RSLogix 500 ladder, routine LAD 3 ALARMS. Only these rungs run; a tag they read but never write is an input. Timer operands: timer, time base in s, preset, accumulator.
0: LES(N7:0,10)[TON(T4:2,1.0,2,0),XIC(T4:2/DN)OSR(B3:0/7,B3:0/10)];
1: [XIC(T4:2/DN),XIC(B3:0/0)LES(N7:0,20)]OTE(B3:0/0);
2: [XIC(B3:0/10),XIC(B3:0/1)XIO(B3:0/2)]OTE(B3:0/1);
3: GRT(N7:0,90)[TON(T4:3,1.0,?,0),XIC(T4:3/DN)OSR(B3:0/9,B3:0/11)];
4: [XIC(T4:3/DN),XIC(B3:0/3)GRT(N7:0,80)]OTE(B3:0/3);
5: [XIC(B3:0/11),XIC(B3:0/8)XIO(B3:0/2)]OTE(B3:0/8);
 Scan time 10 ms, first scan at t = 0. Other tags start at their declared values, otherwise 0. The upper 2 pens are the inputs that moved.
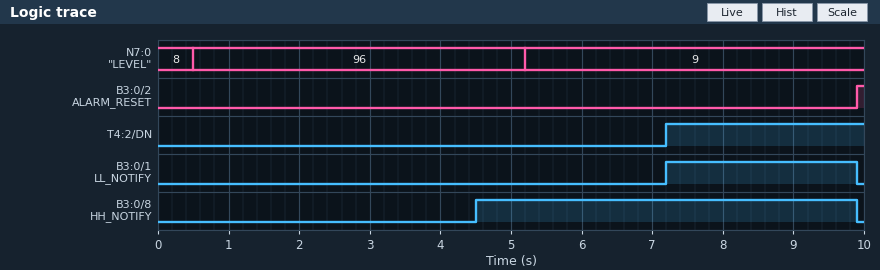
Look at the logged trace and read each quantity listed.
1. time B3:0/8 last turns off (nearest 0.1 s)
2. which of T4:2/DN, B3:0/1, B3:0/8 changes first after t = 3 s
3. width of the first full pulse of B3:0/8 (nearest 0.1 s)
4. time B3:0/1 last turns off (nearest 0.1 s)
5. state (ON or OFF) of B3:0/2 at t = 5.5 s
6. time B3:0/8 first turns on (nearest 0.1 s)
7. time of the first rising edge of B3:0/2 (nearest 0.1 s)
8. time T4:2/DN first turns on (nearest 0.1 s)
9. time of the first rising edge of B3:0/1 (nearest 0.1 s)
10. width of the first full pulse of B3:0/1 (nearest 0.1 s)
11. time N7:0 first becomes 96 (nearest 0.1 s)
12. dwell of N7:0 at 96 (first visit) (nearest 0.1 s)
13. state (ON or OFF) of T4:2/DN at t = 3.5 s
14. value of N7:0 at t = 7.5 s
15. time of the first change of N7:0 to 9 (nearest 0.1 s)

9.9 s
B3:0/8
5.4 s
9.9 s
OFF
4.5 s
9.9 s
7.2 s
7.2 s
2.7 s
0.5 s
4.7 s
OFF
9
5.2 s
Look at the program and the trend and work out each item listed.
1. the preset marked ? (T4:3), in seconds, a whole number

4 s
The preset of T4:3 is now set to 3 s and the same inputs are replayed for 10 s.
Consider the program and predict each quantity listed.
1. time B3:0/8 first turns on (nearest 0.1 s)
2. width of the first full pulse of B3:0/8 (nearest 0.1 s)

3.5 s
6.4 s
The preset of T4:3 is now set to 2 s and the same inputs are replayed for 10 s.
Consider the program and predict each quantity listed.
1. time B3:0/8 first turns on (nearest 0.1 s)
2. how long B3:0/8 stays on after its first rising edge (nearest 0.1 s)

2.5 s
7.4 s
